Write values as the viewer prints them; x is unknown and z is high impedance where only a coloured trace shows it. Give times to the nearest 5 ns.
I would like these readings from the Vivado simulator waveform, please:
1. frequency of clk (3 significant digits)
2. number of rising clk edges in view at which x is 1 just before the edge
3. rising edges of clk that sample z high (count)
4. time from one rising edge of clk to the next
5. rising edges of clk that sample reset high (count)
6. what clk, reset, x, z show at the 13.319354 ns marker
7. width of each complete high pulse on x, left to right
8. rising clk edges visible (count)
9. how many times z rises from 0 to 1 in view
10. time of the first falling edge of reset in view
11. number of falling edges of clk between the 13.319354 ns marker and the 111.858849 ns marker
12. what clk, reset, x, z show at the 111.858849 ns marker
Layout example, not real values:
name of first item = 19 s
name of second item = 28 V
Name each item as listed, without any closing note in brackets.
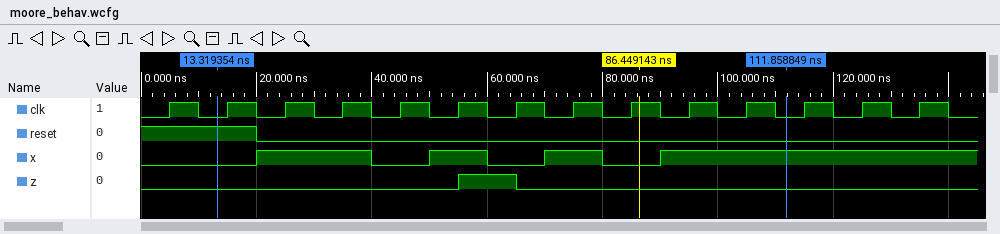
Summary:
frequency of clk = 100 MHz
number of rising clk edges in view at which x is 1 just before the edge = 9
rising edges of clk that sample z high = 1
time from one rising edge of clk to the next = 10 ns
rising edges of clk that sample reset high = 2
what clk, reset, x, z show at the 13.319354 ns marker = clk=0, reset=1, x=0, z=0
width of each complete high pulse on x, left to right = 20 ns, 10 ns, 10 ns
rising clk edges visible = 14
how many times z rises from 0 to 1 in view = 1
time of the first falling edge of reset in view = 20 ns
number of falling edges of clk between the 13.319354 ns marker and the 111.858849 ns marker = 10
what clk, reset, x, z show at the 111.858849 ns marker = clk=0, reset=0, x=1, z=0
